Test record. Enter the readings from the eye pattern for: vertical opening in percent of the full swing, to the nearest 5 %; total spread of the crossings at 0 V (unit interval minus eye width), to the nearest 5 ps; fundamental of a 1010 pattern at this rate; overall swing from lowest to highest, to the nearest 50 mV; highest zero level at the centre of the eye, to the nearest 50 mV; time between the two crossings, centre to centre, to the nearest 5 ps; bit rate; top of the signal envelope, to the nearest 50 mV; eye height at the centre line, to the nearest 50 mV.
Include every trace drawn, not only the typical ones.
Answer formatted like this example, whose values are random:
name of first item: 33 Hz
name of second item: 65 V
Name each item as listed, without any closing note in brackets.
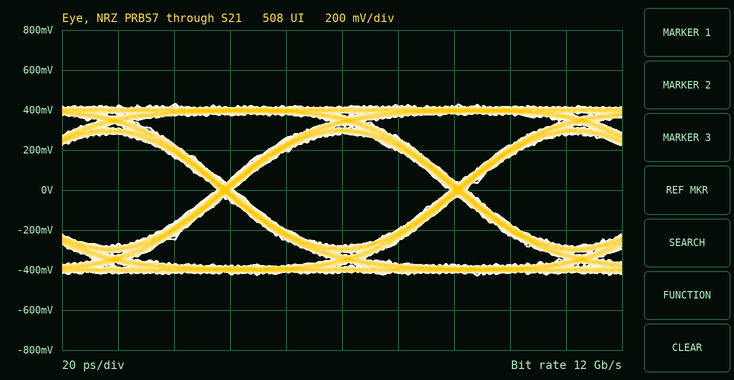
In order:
vertical opening in percent of the full swing, to the nearest 5 %: 65 %
total spread of the crossings at 0 V (unit interval minus eye width), to the nearest 5 ps: 5 ps
fundamental of a 1010 pattern at this rate: 6 GHz
overall swing from lowest to highest, to the nearest 50 mV: 850 mV
highest zero level at the centre of the eye, to the nearest 50 mV: -300 mV
time between the two crossings, centre to centre, to the nearest 5 ps: 85 ps
bit rate: 12 Gb/s
top of the signal envelope, to the nearest 50 mV: 450 mV
eye height at the centre line, to the nearest 50 mV: 550 mV
